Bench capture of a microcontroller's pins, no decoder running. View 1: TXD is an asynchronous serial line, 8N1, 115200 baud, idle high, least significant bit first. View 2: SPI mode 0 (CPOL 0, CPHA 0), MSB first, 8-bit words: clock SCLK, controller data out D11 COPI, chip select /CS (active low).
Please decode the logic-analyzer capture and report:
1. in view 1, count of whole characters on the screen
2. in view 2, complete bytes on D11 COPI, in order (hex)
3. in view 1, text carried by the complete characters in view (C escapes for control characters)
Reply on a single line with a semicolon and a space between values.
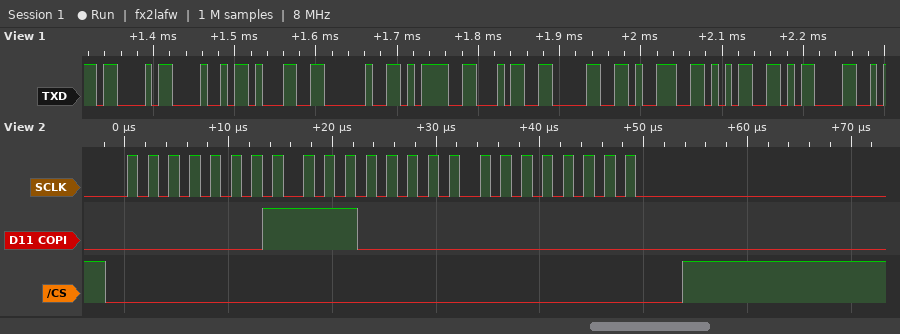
10; 0x01 0xE0 0x00; "CH1 =4095\r"
